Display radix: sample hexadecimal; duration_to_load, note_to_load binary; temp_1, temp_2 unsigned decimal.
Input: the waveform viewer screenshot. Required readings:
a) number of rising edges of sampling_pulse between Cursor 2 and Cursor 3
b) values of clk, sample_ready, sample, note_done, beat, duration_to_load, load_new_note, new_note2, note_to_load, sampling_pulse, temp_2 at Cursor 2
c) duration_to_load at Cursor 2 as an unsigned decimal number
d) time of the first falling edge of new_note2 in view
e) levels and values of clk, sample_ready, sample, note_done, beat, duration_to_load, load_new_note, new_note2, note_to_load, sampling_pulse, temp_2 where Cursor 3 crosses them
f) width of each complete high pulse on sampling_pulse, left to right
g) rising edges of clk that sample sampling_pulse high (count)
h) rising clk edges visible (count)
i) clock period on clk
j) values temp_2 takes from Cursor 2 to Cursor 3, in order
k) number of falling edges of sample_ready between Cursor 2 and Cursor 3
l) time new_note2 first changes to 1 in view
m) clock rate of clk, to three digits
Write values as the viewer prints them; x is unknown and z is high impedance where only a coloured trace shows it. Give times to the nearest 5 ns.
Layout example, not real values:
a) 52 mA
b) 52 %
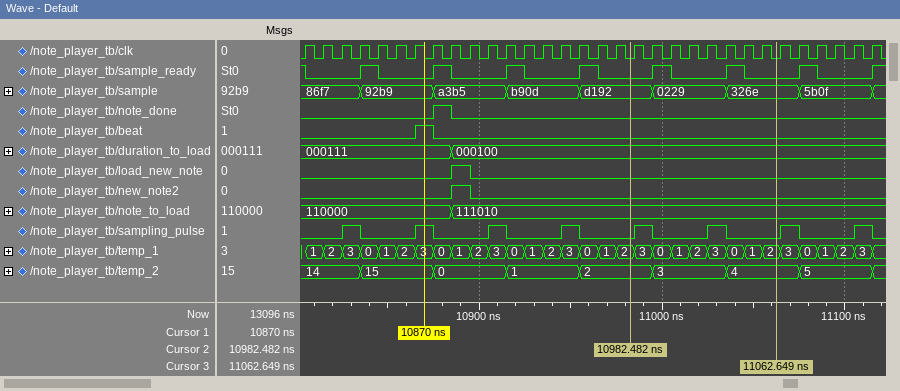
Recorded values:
a) 2
b) clk=0, sample_ready=0, sample=d192, note_done=0, beat=0, duration_to_load=000100, load_new_note=0, new_note2=0, note_to_load=111010, sampling_pulse=0, temp_2=2
c) 4
d) 10895 ns
e) clk=0, sample_ready=0, sample=326e, note_done=0, beat=0, duration_to_load=000100, load_new_note=0, new_note2=0, note_to_load=111010, sampling_pulse=0, temp_2=4
f) 10 ns, 10 ns, 10 ns, 10 ns, 10 ns, 10 ns, 10 ns, 10 ns
g) 8
h) 32
i) 10 ns
j) 2, 3, 4
k) 2
l) 10885 ns
m) 100 MHz
